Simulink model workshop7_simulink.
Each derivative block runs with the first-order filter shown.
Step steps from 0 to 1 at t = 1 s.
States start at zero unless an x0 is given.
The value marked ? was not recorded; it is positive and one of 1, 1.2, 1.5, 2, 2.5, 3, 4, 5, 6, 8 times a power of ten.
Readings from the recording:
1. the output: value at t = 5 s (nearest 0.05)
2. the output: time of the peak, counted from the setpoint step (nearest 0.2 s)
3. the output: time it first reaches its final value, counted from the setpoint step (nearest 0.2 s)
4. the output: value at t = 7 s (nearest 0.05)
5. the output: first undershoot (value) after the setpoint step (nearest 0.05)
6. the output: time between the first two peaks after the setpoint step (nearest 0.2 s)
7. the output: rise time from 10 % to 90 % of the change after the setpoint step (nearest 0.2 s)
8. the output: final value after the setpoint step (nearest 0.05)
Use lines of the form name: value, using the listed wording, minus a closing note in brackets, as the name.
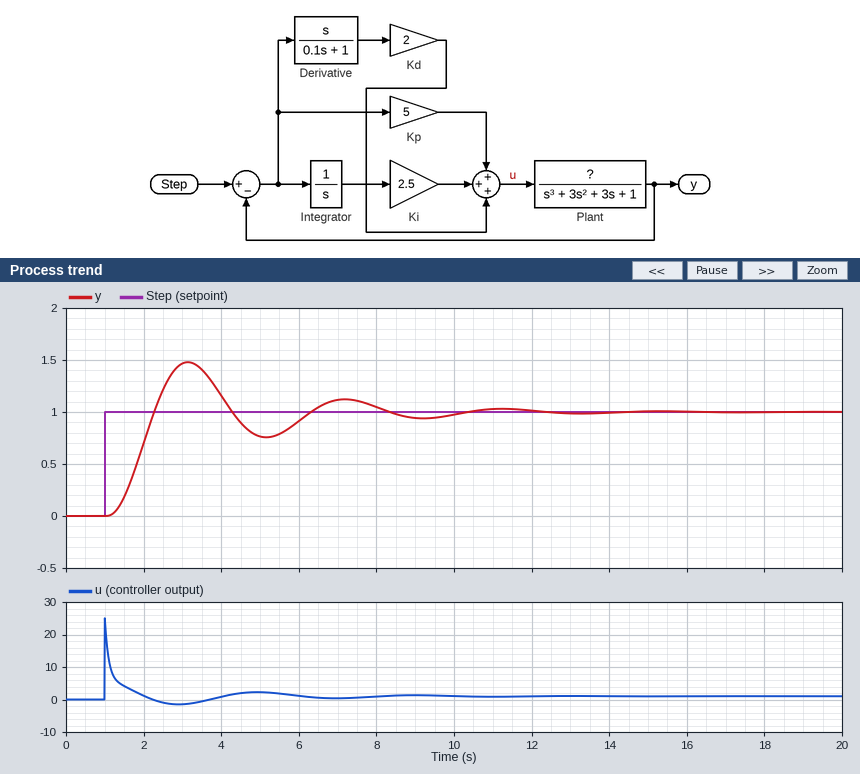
the output: value at t = 5 s: 0.75
the output: time of the peak, counted from the setpoint step: 2.2 s
the output: time it first reaches its final value, counted from the setpoint step: 1.2 s
the output: value at t = 7 s: 1.10
the output: first undershoot (value) after the setpoint step: 0.75
the output: time between the first two peaks after the setpoint step: 4.0 s
the output: rise time from 10 % to 90 % of the change after the setpoint step: 0.8 s
the output: final value after the setpoint step: 1.00
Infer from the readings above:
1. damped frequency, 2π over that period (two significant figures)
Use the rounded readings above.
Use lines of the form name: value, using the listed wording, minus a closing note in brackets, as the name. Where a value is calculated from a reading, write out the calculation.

damped frequency, 2π over that period: 2π / 4 = 1.6 rad/s
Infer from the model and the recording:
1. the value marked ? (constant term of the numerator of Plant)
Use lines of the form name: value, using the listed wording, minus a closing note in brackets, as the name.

the value marked ?: 1
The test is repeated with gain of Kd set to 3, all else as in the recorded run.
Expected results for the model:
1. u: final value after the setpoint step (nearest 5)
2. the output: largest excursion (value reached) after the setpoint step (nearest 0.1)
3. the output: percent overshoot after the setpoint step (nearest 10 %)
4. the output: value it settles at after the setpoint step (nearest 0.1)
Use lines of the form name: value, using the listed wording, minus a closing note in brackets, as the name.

u: final value after the setpoint step: 0
the output: largest excursion (value reached) after the setpoint step: 1.4
the output: percent overshoot after the setpoint step: 40 %
the output: value it settles at after the setpoint step: 1.0
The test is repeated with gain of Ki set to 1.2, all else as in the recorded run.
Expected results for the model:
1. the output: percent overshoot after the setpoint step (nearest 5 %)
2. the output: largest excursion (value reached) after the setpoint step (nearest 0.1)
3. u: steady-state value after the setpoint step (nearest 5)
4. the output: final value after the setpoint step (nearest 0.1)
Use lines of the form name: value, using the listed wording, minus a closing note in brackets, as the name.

the output: percent overshoot after the setpoint step: 30 %
the output: largest excursion (value reached) after the setpoint step: 1.3
u: steady-state value after the setpoint step: 0
the output: final value after the setpoint step: 1.0
